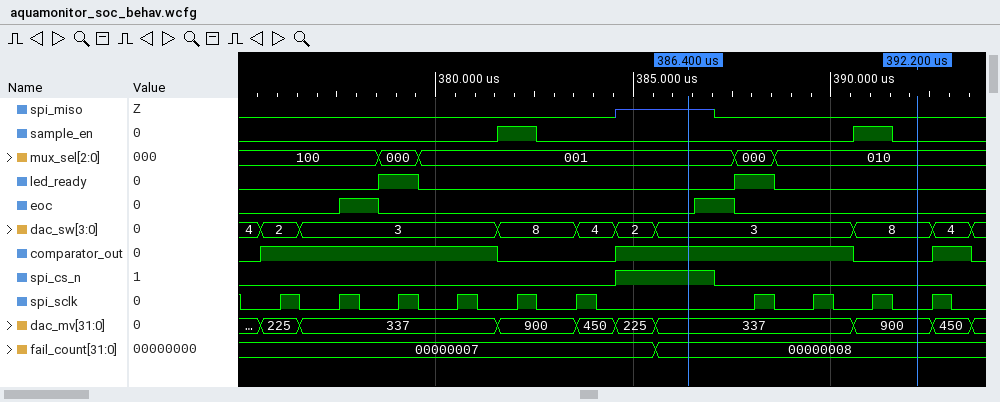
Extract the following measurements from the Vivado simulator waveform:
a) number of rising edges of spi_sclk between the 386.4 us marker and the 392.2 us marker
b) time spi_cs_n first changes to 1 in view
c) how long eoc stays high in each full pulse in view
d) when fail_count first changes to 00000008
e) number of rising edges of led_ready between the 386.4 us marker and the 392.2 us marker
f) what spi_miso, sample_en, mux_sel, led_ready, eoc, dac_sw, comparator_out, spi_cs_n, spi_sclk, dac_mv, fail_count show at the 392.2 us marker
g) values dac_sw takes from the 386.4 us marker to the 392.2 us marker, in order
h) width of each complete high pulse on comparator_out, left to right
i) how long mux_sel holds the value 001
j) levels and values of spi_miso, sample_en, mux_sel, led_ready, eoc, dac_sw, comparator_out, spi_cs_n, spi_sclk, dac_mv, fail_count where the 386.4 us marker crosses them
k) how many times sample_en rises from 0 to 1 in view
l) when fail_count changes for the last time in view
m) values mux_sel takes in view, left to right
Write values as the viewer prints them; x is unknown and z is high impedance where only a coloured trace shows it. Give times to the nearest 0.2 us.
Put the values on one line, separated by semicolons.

3; 384.6 us; 1 us, 1 us; 385.6 us; 1; spi_miso=0, sample_en=0, mux_sel=010, led_ready=0, eoc=0, dac_sw=8, comparator_out=0, spi_cs_n=0, spi_sclk=0, dac_mv=900, fail_count=00000008; 3, 8; 6 us, 6 us, 1 us; 8 us; spi_miso=z, sample_en=0, mux_sel=001, led_ready=0, eoc=0, dac_sw=3, comparator_out=1, spi_cs_n=1, spi_sclk=0, dac_mv=337, fail_count=00000008; 2; 385.6 us; 100, 000, 001, 000, 010
